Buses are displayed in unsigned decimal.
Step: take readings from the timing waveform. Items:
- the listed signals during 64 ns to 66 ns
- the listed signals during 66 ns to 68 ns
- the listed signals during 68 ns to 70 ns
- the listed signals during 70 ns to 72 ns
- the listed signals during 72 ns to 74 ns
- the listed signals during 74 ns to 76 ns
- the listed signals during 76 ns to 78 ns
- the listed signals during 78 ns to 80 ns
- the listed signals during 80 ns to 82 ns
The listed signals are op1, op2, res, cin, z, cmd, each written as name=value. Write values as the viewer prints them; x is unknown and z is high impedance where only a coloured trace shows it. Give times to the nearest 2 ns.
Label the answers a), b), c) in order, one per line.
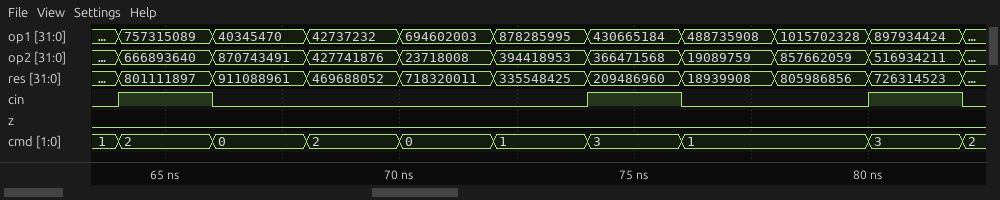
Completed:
a) op1=757315089, op2=666893640, res=801111897, cin=1, z=0, cmd=2
b) op1=40345470, op2=870743491, res=911088961, cin=0, z=0, cmd=0
c) op1=42737232, op2=427741876, res=469688052, cin=0, z=0, cmd=2
d) op1=694602003, op2=23718008, res=718320011, cin=0, z=0, cmd=0
e) op1=878285995, op2=394418953, res=335548425, cin=0, z=0, cmd=1
f) op1=430665184, op2=366471568, res=209486960, cin=1, z=0, cmd=3
g) op1=488735908, op2=19089759, res=18939908, cin=0, z=0, cmd=1
h) op1=1015702328, op2=857662059, res=805986856, cin=0, z=0, cmd=1
i) op1=897934424, op2=516934211, res=726314523, cin=1, z=0, cmd=3
